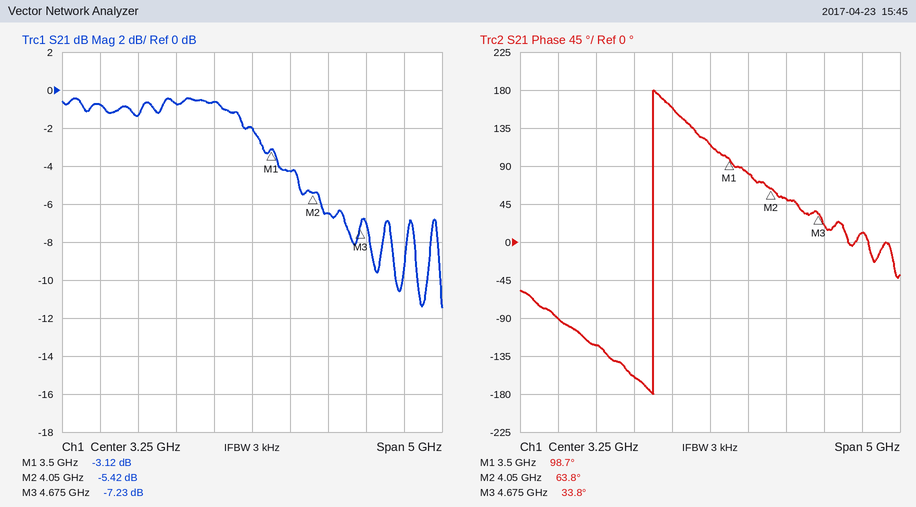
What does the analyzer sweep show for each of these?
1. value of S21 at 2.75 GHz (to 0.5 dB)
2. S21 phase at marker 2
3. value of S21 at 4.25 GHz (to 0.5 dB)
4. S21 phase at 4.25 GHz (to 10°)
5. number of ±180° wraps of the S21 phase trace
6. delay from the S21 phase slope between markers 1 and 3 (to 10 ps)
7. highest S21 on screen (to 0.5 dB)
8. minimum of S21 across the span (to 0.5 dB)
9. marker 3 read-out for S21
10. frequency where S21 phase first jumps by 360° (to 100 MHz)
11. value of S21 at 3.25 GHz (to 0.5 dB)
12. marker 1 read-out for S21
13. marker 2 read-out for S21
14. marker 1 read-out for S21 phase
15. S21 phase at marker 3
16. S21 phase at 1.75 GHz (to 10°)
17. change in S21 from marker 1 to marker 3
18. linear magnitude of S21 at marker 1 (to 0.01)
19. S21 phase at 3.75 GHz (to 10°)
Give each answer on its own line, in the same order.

-0.5 dB
63.8°
-6.5 dB
50°
1
150 ps
-0.5 dB
-11.5 dB
-7.23 dB
2.5 GHz
-2.0 dB
-3.12 dB
-5.42 dB
98.7°
33.8°
-120°
-4.11 dB
0.70
80°
